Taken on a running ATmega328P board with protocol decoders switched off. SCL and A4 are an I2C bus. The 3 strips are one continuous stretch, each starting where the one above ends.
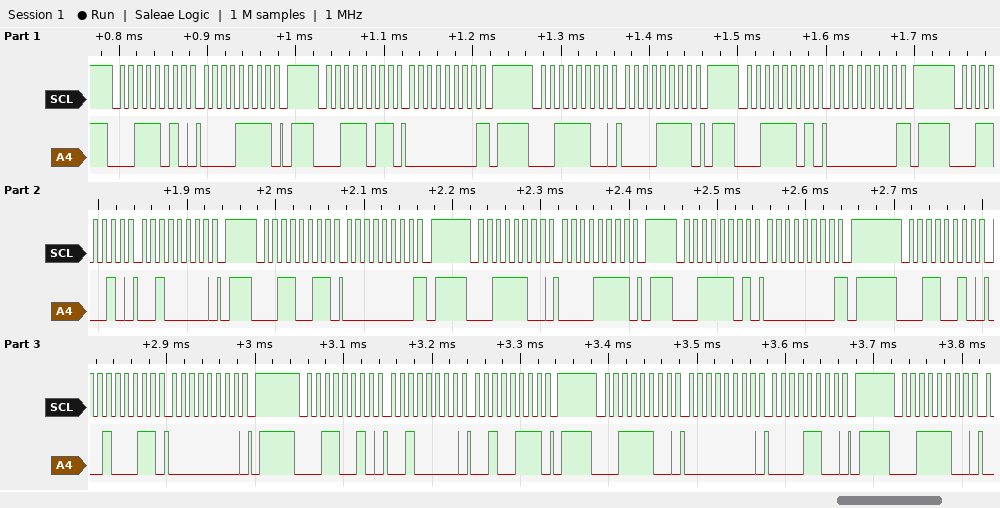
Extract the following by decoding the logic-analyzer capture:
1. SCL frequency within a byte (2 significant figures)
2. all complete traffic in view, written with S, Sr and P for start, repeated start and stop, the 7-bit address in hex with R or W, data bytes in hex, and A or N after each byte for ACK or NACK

100 kHz
S 1DW A 0F A P S 1DR A 00 N P S 1EW A 0F A P S 1ER A 00 N P S 19W A 20 A P S 19R A 00 N P S 1EW A 0F A P S 1ER A 00 N P S 19W A 23 A 00 A P S 19W A 20 A 27 A P S 1EW A 00 A 0C A P S 1EW A
